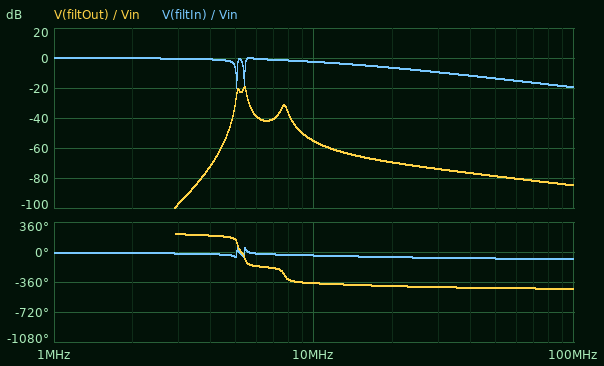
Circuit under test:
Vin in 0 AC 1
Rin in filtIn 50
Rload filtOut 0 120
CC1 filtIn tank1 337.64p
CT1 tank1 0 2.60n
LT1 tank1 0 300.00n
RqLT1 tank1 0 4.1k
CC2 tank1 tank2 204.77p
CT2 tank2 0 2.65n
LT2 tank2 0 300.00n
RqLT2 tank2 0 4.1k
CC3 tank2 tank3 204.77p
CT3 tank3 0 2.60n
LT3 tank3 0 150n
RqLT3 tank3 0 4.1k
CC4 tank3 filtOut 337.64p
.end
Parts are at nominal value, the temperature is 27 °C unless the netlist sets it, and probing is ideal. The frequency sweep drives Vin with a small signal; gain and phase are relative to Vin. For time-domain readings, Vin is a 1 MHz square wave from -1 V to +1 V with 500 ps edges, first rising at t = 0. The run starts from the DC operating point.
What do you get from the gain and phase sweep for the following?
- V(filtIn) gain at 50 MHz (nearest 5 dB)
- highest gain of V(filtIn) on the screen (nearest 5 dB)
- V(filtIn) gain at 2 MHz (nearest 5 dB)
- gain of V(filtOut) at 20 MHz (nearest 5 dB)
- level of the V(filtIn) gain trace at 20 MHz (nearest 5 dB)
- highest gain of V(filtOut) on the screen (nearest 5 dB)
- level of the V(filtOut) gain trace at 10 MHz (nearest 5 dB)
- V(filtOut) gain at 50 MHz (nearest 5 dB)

-15 dB
0 dB
0 dB
-70 dB
-5 dB
-20 dB
-55 dB
-80 dB
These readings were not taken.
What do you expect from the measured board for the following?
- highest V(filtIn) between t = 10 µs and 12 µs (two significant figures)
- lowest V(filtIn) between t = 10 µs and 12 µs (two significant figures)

1.2 V
-1.2 V
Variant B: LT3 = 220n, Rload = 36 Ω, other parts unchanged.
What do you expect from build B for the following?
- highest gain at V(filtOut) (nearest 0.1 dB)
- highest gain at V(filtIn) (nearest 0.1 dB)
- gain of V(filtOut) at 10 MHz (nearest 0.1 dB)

-16.4 dB
0 dB
-63.3 dB
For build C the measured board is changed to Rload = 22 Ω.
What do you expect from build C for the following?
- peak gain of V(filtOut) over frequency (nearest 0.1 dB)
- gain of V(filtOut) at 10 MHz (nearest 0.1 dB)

-29.0 dB
-63.9 dB
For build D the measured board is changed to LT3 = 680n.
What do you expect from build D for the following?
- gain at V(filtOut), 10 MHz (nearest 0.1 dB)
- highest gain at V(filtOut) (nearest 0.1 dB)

-62.1 dB
-13.9 dB
